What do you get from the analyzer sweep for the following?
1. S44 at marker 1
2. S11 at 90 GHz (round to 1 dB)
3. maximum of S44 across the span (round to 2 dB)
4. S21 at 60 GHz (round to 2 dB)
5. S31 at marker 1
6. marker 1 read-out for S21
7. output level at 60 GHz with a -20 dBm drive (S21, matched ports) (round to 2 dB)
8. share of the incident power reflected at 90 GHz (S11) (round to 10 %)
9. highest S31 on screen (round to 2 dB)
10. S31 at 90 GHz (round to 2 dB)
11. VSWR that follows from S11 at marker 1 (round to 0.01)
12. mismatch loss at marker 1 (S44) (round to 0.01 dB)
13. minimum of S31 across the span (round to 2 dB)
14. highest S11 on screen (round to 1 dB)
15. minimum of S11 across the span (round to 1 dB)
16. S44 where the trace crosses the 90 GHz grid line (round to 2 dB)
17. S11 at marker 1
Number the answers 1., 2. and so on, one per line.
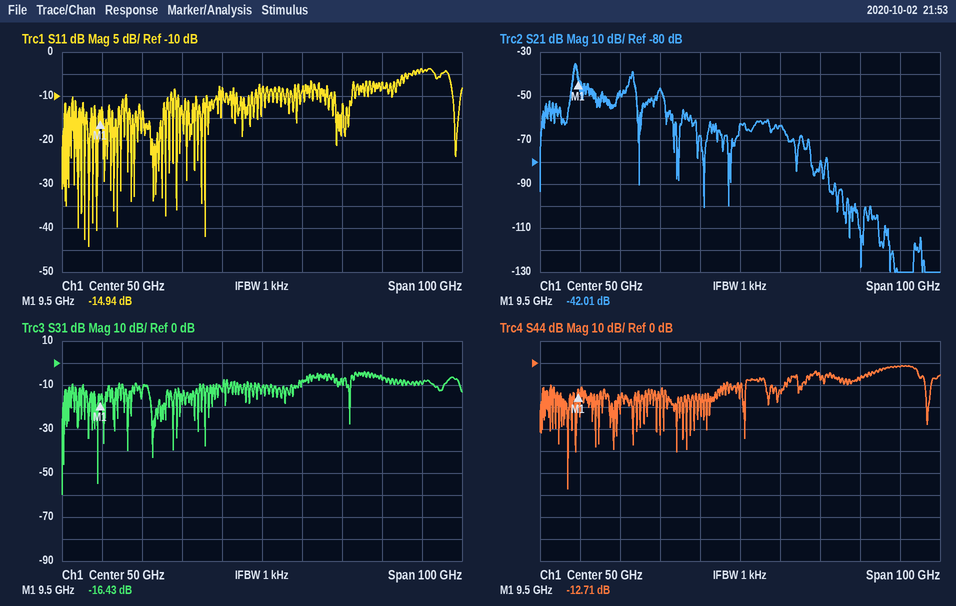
1. -12.71 dB
2. -4 dB
3. -2 dB
4. -64 dB
5. -16.43 dB
6. -42.01 dB
7. -84 dBm
8. 40 %
9. -4 dB
10. -10 dB
11. 1.44
12. 0.24 dB
13. -60 dB
14. -4 dB
15. -44 dB
16. -2 dB
17. -14.94 dB
